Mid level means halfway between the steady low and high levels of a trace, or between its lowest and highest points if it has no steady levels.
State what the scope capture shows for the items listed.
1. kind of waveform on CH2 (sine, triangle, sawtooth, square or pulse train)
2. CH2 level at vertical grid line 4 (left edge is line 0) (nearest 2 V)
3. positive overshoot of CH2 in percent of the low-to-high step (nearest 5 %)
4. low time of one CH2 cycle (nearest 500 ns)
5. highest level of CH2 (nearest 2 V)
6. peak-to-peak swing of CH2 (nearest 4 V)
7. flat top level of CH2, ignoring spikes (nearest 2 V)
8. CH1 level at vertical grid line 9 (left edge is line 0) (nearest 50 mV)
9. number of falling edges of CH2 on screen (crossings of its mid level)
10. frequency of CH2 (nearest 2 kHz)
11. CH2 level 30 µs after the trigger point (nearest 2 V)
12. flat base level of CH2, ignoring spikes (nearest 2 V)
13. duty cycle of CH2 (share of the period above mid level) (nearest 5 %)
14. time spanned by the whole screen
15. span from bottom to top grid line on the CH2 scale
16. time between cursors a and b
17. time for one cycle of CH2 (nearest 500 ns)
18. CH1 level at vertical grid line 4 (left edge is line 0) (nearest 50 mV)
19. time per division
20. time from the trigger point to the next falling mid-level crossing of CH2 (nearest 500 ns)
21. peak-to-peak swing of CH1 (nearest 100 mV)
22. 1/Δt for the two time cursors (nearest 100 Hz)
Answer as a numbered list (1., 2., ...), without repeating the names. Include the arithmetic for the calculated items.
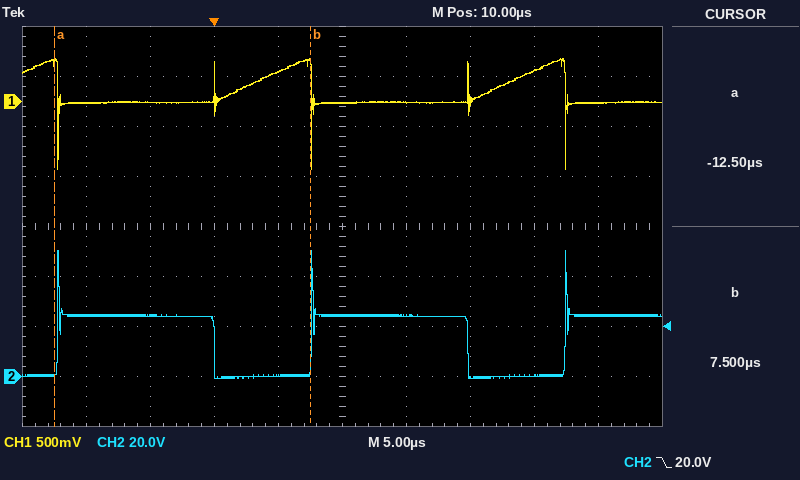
1. pulse train
2. 0 V
3. 105 %
4. 7.5 µs
5. 50 V
6. 52 V
7. 24 V
8. 0 mV
9. 2
10. 1 / 20.0 µs ≈ 50 kHz
11. 24 V
12. 0 V
13. 60 %
14. 50 µs
15. 160 V
16. 7.5 µs − (-12.5 µs) = 20.0 µs
17. 20.0 µs
18. 300 mV
19. 5 µs
20. 20.0 µs
21. 1.10 V
22. 1 / 20.0 µs ≈ 50.0 kHz
